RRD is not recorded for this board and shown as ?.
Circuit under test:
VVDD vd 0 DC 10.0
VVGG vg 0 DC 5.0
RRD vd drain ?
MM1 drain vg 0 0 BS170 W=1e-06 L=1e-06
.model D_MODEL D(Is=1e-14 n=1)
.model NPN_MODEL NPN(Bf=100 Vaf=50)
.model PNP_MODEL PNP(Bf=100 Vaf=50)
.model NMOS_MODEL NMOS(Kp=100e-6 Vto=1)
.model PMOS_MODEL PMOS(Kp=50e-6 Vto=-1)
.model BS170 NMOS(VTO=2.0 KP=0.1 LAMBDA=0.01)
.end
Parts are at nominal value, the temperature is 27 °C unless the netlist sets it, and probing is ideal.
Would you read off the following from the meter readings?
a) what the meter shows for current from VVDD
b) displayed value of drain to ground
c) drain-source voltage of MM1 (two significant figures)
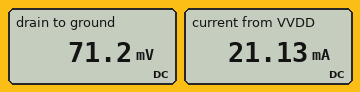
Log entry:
21.13 mA
71.2 mV
71 mV
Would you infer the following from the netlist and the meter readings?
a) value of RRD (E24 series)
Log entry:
470 Ω
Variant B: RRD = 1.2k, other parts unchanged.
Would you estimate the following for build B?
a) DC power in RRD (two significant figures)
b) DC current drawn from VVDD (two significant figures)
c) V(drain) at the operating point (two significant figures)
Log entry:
83 mW
8.3 mA
28 mV
